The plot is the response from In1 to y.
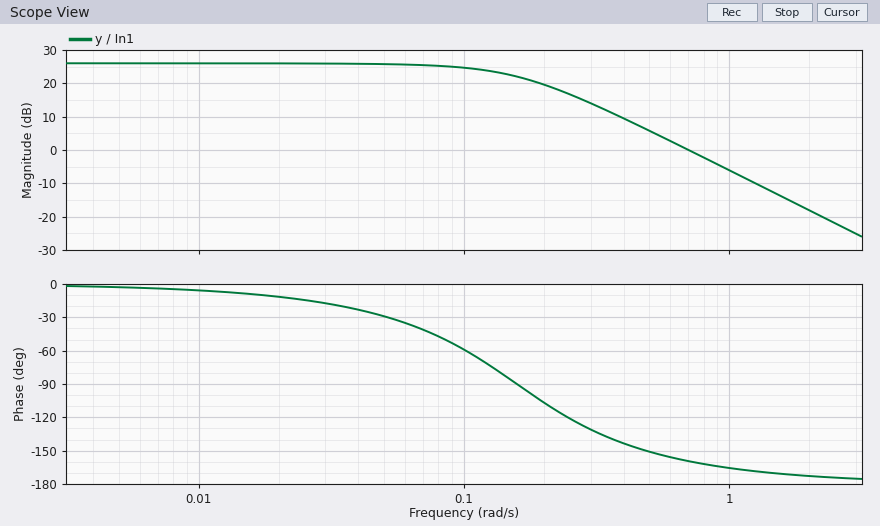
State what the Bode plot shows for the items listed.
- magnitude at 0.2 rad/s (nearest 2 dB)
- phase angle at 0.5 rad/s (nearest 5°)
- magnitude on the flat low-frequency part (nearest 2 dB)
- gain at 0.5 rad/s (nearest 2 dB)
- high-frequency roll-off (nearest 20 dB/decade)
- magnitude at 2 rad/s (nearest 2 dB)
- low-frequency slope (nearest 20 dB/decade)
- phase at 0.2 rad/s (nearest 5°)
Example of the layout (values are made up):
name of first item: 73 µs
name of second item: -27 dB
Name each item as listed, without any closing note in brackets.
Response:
magnitude at 0.2 rad/s: 20 dB
phase angle at 0.5 rad/s: -150°
magnitude on the flat low-frequency part: 26 dB
gain at 0.5 rad/s: 6 dB
high-frequency roll-off: -40 dB/decade
magnitude at 2 rad/s: -18 dB
low-frequency slope: 0 dB/decade
phase at 0.2 rad/s: -105°
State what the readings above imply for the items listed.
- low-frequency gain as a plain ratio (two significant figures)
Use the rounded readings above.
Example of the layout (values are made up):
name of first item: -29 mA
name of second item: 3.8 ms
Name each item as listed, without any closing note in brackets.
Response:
low-frequency gain as a plain ratio: 20
